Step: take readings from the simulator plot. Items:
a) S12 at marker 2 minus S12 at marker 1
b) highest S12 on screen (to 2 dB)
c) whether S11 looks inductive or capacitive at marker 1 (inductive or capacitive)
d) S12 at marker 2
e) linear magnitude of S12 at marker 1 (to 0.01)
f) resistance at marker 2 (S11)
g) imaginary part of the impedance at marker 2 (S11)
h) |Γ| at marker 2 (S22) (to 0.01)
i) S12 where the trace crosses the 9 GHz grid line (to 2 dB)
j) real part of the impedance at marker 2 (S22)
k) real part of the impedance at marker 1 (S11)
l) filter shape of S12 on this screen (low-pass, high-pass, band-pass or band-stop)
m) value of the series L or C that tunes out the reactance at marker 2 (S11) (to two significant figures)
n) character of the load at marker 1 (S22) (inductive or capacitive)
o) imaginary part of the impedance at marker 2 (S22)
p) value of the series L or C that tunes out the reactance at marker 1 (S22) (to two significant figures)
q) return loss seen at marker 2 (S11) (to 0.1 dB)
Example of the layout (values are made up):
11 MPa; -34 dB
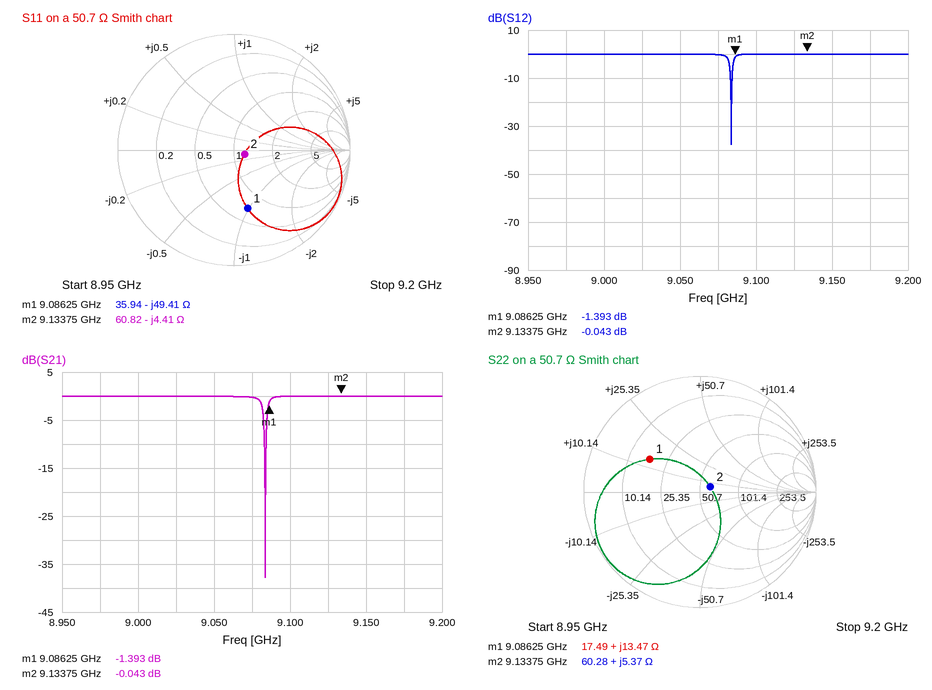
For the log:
1.350 dB; 0 dB; capacitive; -0.043 dB; 0.85; 60.82 Ω; -4.41 Ω; 0.10; 0 dB; 60.28 Ω; 35.94 Ω; band-stop; 77 pH; inductive; +5.37 Ω; 1.3 pF; 20.1 dB
